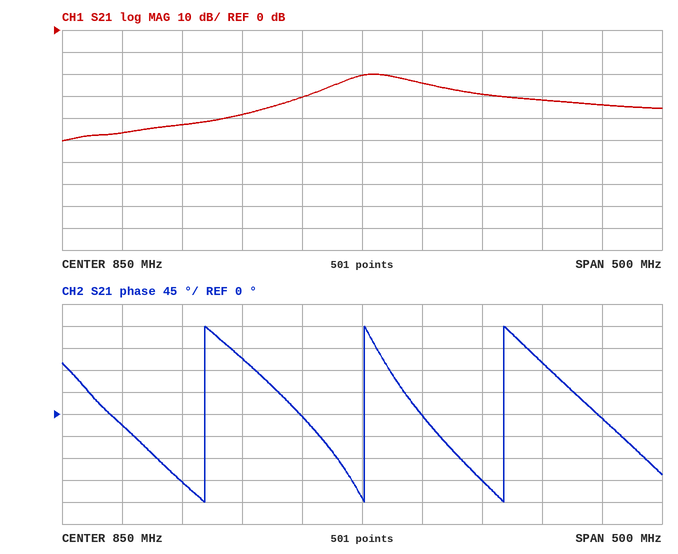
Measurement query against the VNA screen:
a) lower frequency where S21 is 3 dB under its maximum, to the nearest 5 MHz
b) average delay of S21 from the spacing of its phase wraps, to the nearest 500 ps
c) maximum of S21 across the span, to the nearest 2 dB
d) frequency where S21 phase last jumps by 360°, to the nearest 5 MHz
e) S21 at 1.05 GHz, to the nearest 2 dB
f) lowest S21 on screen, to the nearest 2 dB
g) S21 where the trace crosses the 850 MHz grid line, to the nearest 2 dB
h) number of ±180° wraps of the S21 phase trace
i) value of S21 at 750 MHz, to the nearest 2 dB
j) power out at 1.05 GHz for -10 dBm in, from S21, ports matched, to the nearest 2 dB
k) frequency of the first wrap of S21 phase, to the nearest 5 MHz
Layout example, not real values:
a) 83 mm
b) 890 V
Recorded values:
a) 835 MHz
b) 8.0 ns
c) -20 dB
d) 970 MHz
e) -34 dB
f) -50 dB
g) -20 dB
h) 3
i) -38 dB
j) -44 dBm
k) 720 MHz
